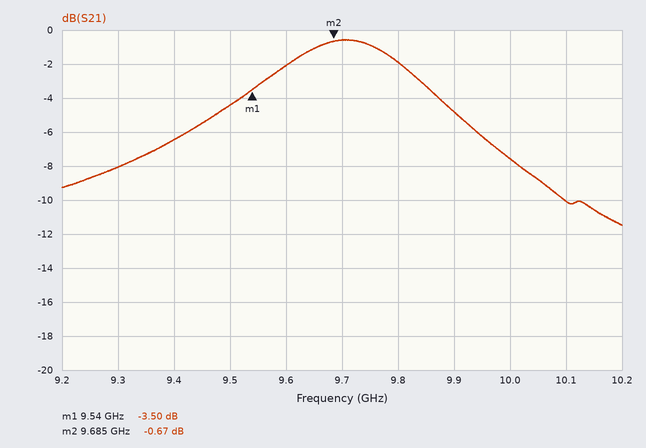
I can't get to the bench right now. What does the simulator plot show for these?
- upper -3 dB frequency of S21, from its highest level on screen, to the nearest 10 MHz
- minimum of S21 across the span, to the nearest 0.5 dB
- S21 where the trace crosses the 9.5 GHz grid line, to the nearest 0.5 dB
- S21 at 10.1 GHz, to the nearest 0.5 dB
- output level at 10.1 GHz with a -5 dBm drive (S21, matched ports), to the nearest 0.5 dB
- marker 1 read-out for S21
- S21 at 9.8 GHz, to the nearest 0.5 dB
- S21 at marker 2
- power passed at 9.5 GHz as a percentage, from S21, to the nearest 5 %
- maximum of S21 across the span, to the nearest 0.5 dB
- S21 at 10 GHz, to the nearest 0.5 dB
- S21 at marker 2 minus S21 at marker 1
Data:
9.86 GHz
-11.5 dB
-4.5 dB
-10.0 dB
-15.0 dBm
-3.50 dB
-2.0 dB
-0.67 dB
35 %
-0.5 dB
-7.5 dB
2.83 dB
